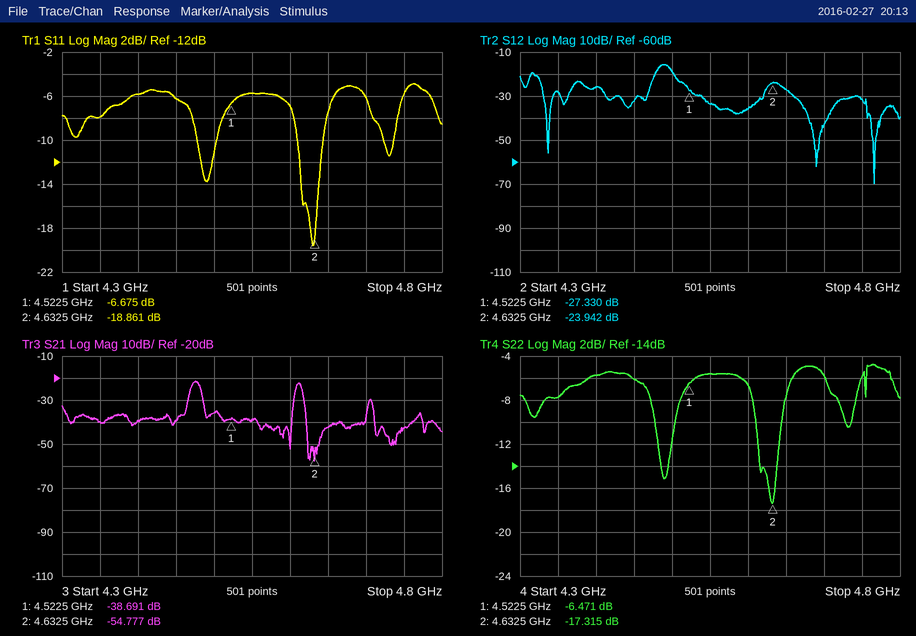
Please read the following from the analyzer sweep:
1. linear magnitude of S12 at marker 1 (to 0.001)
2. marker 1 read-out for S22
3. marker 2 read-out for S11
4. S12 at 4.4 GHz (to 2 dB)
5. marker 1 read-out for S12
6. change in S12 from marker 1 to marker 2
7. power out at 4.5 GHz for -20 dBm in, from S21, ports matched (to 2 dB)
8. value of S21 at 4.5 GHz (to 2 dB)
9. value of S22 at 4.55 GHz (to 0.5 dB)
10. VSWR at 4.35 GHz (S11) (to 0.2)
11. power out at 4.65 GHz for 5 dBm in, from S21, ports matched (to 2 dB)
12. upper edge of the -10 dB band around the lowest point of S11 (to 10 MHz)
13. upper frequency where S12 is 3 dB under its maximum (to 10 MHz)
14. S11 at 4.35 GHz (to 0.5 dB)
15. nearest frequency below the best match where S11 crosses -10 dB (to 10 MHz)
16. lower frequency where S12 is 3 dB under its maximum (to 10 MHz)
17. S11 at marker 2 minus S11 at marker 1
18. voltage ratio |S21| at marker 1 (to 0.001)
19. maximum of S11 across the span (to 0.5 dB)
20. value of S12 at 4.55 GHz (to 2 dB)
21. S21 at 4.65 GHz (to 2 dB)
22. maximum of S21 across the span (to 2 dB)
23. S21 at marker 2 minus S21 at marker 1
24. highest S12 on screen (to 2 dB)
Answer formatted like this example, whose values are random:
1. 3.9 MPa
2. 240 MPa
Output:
1. 0.043
2. -6.471 dB
3. -18.861 dB
4. -26 dB
5. -27.330 dB
6. 3.388 dB
7. -56 dBm
8. -36 dB
9. -5.5 dB
10. 2.4
11. -38 dBm
12. 4.64 GHz
13. 4.50 GHz
14. -8.0 dB
15. 4.61 GHz
16. 4.48 GHz
17. -12.186 dB
18. 0.012
19. -5.0 dB
20. -34 dB
21. -42 dB
22. -22 dB
23. -16.086 dB
24. -16 dB
